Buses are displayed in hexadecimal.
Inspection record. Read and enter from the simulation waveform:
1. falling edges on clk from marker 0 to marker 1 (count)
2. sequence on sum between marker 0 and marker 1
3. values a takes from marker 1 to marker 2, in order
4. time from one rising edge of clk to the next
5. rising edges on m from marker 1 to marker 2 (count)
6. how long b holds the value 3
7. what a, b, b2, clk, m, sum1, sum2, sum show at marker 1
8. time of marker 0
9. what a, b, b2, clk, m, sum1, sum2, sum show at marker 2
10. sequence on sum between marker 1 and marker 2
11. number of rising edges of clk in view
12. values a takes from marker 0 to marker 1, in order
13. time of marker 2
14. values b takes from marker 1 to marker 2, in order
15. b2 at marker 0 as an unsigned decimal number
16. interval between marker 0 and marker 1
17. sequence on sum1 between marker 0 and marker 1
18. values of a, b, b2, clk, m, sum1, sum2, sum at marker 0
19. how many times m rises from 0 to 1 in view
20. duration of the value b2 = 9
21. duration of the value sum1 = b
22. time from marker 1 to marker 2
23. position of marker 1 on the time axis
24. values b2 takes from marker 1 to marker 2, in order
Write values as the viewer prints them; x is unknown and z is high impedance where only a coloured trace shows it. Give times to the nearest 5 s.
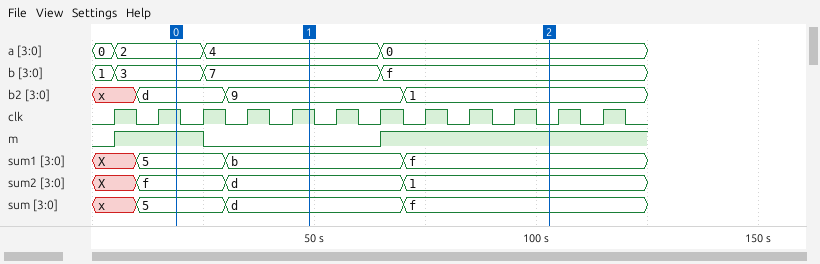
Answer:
3
5, d
4, 0
10 s
1
20 s
a=4, b=7, b2=9, clk=1, m=0, sum1=b, sum2=d, sum=d
20 s
a=0, b=f, b2=1, clk=0, m=1, sum1=f, sum2=1, sum=f
d, f
12
2, 4
105 s
7, f
13
30 s
5, b
a=2, b=3, b2=d, clk=1, m=1, sum1=5, sum2=f, sum=5
2
40 s
40 s
55 s
50 s
9, 1
